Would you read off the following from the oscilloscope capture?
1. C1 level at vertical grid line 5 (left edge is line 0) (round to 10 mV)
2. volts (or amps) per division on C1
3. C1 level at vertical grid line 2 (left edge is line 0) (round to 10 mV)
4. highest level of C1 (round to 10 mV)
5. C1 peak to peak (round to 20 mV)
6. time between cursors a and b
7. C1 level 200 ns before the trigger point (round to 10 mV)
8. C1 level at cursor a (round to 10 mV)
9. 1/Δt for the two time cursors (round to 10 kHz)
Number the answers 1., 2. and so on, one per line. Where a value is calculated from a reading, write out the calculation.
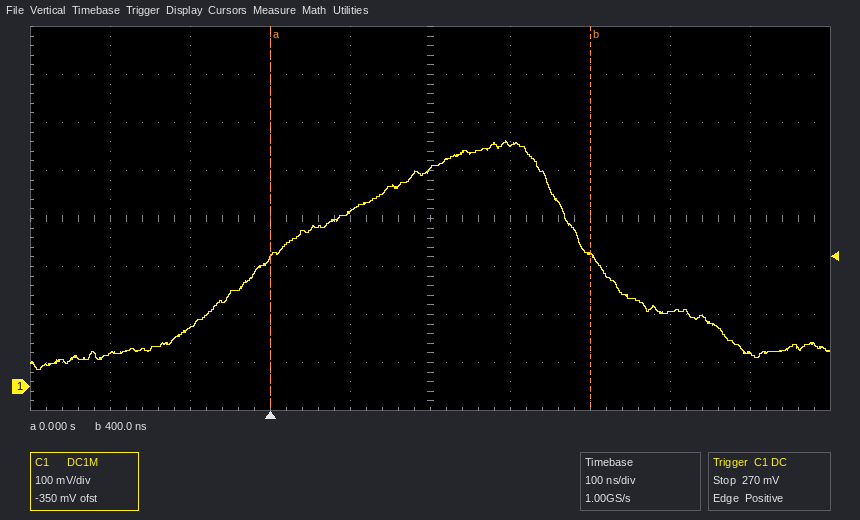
1. 450 mV
2. 100 mV
3. 120 mV
4. 510 mV
5. 480 mV
6. 400 ns − (0 s) = 400 ns
7. 70 mV
8. 270 mV
9. 1 / 400 ns ≈ 2.50 MHz
